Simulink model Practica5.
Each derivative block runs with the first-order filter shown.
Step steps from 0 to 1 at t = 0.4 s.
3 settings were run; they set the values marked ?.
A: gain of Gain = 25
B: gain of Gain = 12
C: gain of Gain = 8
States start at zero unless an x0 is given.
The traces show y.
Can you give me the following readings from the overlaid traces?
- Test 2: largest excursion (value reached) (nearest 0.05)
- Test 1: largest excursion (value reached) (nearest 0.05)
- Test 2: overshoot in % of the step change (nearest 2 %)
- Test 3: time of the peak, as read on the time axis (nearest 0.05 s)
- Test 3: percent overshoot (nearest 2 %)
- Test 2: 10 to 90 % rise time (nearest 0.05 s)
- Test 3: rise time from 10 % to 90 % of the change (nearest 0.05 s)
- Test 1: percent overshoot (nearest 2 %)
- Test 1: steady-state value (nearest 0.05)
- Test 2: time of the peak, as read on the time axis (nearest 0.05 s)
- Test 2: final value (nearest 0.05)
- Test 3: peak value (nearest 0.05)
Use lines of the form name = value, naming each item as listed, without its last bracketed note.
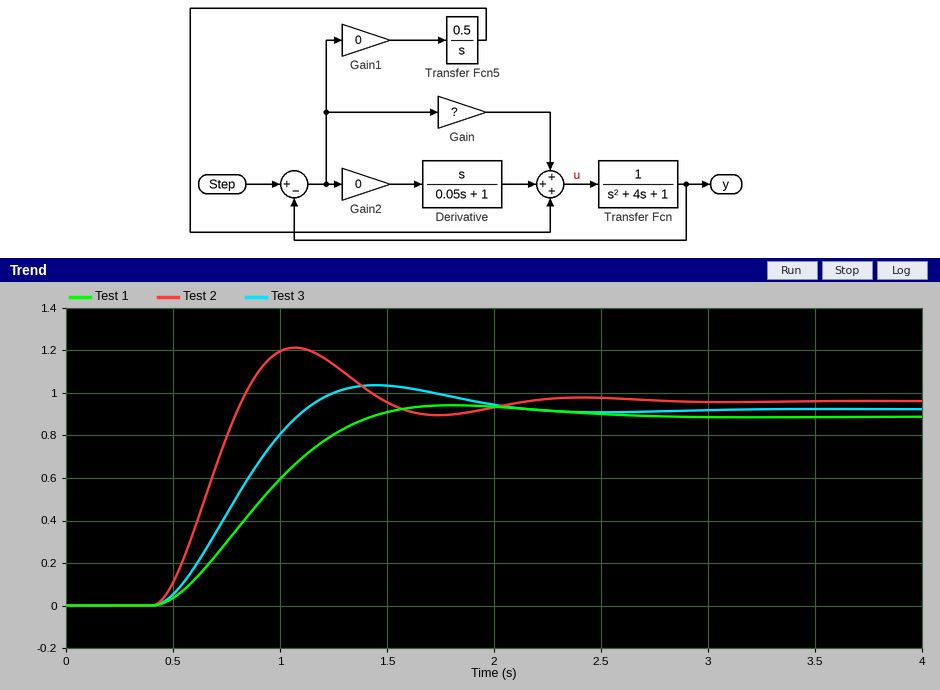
Test 2: largest excursion (value reached) = 1.20
Test 1: largest excursion (value reached) = 0.95
Test 2: overshoot in % of the step change = 26 %
Test 3: time of the peak, as read on the time axis = 1.45 s
Test 3: percent overshoot = 12 %
Test 2: 10 to 90 % rise time = 0.30 s
Test 3: rise time from 10 % to 90 % of the change = 0.50 s
Test 1: percent overshoot = 6 %
Test 1: steady-state value = 0.90
Test 2: time of the peak, as read on the time axis = 1.05 s
Test 2: final value = 0.95
Test 3: peak value = 1.05
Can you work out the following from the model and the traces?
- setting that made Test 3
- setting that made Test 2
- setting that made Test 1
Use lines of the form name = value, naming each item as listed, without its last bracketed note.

setting that made Test 3 = B
setting that made Test 2 = A
setting that made Test 1 = C
